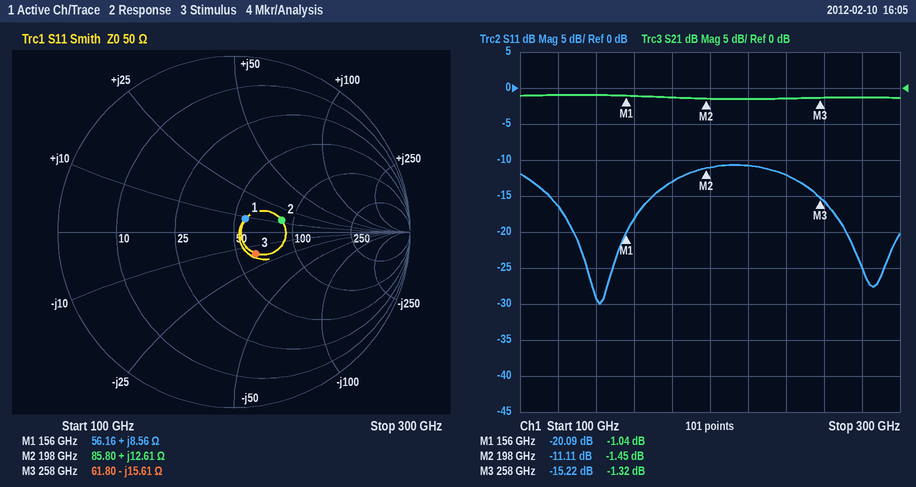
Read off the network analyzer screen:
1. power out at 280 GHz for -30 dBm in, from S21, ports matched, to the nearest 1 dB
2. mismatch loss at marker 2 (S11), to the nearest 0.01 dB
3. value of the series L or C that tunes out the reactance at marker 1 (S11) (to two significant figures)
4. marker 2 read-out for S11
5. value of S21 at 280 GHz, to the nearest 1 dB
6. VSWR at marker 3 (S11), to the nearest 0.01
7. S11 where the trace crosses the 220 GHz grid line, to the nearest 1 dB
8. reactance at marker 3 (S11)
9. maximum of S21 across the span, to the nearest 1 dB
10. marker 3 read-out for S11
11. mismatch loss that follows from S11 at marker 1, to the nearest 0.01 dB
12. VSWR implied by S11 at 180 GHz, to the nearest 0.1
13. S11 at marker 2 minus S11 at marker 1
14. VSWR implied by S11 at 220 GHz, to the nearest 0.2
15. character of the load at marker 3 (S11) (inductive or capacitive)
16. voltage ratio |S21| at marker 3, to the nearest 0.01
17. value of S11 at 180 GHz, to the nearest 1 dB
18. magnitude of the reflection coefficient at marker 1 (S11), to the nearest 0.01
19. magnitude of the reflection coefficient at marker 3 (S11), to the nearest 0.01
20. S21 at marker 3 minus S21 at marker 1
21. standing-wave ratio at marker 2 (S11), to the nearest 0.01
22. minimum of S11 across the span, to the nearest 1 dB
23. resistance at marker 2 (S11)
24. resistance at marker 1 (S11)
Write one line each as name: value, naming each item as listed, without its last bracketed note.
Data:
power out at 280 GHz for -30 dBm in, from S21, ports matched, to the nearest 1 dB: -31 dBm
mismatch loss at marker 2 (S11), to the nearest 0.01 dB: 0.35 dB
value of the series L or C that tunes out the reactance at marker 1 (S11): 120 fF
marker 2 read-out for S11: -11.11 dB
value of S21 at 280 GHz, to the nearest 1 dB: -1 dB
VSWR at marker 3 (S11), to the nearest 0.01: 1.42
S11 where the trace crosses the 220 GHz grid line, to the nearest 1 dB: -11 dB
reactance at marker 3: -15.61 Ω
maximum of S21 across the span, to the nearest 1 dB: -1 dB
marker 3 read-out for S11: -15.22 dB
mismatch loss that follows from S11 at marker 1, to the nearest 0.01 dB: 0.04 dB
VSWR implied by S11 at 180 GHz, to the nearest 0.1: 1.6
S11 at marker 2 minus S11 at marker 1: 8.98 dB
VSWR implied by S11 at 220 GHz, to the nearest 0.2: 1.8
character of the load at marker 3 (S11): capacitive
voltage ratio |S21| at marker 3, to the nearest 0.01: 0.86
value of S11 at 180 GHz, to the nearest 1 dB: -13 dB
magnitude of the reflection coefficient at marker 1 (S11), to the nearest 0.01: 0.10
magnitude of the reflection coefficient at marker 3 (S11), to the nearest 0.01: 0.17
S21 at marker 3 minus S21 at marker 1: -0.28 dB
standing-wave ratio at marker 2 (S11), to the nearest 0.01: 1.77
minimum of S11 across the span, to the nearest 1 dB: -30 dB
resistance at marker 2: 85.80 Ω
resistance at marker 1: 56.16 Ω
